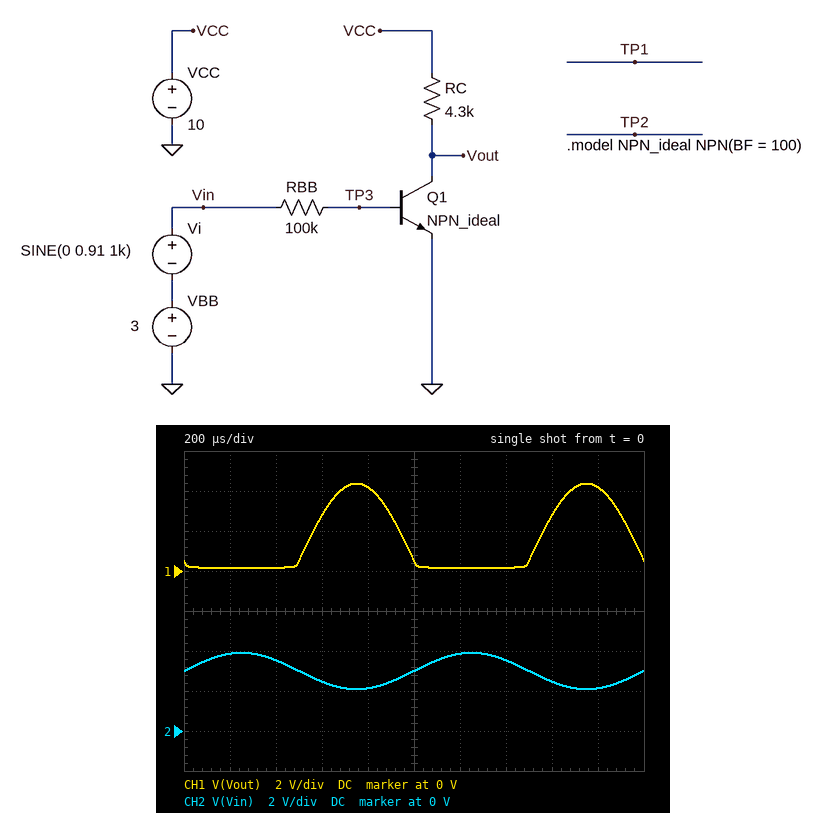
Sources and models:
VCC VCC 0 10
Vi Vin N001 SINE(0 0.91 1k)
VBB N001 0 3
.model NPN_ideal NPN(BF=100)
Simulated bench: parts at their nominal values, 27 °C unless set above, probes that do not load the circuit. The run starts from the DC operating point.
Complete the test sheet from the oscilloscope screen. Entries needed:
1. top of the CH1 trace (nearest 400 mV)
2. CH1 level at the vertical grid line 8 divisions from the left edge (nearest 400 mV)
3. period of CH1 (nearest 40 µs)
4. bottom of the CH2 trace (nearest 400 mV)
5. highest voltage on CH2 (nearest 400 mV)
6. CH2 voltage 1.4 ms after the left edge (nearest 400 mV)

4.4 V
2.8 V
1.00 ms
2.0 V
4.0 V
3.6 V
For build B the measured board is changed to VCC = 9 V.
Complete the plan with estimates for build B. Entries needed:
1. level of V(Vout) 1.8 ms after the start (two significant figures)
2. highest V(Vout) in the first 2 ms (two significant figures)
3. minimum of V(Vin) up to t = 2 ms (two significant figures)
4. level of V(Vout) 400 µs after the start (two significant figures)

3.2 V
3.4 V
2.1 V
150 mV
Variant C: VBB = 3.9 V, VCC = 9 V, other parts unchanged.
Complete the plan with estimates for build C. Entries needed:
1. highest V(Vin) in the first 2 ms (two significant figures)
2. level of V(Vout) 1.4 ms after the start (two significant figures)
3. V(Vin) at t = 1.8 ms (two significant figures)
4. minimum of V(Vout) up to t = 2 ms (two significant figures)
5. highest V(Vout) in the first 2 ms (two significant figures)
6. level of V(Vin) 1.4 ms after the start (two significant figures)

4.8 V
130 mV
3.0 V
120 mV
190 mV
4.4 V
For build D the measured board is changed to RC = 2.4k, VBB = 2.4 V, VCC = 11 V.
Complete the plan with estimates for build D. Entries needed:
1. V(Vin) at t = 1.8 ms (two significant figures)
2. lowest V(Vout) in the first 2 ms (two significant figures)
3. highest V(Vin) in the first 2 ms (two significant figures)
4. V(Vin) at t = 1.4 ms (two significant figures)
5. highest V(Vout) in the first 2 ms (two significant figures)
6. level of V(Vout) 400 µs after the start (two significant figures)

1.5 V
5.0 V
3.3 V
2.9 V
9.3 V
5.9 V
